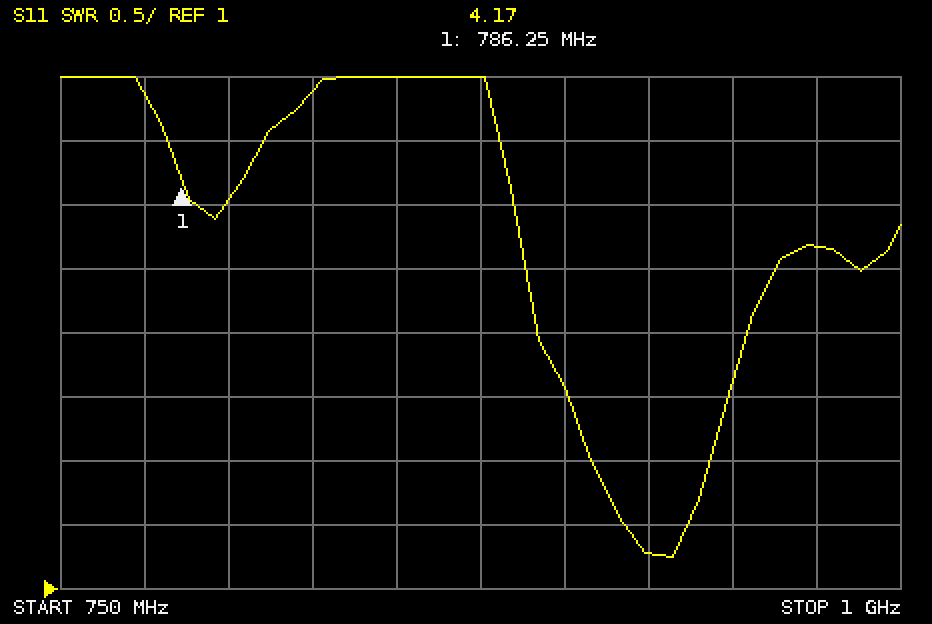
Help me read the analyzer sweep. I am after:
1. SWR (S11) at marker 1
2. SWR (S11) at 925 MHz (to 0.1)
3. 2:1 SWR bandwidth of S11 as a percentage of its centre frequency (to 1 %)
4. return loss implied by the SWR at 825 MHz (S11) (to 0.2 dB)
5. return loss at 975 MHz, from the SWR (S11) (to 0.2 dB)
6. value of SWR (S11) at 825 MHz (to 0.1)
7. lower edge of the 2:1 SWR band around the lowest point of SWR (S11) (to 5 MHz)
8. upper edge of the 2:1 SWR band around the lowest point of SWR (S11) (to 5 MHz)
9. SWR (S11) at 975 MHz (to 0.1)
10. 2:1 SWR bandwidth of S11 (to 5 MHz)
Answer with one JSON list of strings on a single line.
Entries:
["4.17", "1.3", "4 %", "3.6 dB", "4.8 dB", "4.9", "910 MHz", "945 MHz", "3.7", "35 MHz"]
